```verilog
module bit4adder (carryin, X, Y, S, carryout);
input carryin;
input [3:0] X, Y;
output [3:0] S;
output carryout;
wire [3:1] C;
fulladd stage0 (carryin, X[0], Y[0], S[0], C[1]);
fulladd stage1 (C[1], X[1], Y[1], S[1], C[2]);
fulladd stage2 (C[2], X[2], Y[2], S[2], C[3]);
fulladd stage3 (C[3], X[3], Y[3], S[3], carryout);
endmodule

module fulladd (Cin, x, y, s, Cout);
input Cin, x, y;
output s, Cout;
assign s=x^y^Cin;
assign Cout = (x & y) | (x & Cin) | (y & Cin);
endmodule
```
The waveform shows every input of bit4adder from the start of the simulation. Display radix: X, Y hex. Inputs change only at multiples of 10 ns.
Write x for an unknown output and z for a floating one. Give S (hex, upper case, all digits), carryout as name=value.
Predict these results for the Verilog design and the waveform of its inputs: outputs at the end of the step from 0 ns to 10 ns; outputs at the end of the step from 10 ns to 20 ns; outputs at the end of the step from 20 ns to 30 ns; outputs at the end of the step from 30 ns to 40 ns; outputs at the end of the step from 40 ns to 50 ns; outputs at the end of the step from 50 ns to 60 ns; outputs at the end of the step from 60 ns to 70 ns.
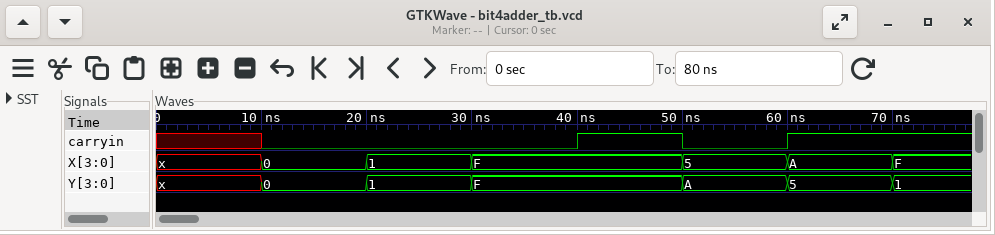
S=x, carryout=x
S=0, carryout=0
S=2, carryout=0
S=E, carryout=1
S=F, carryout=1
S=F, carryout=0
S=0, carryout=1
